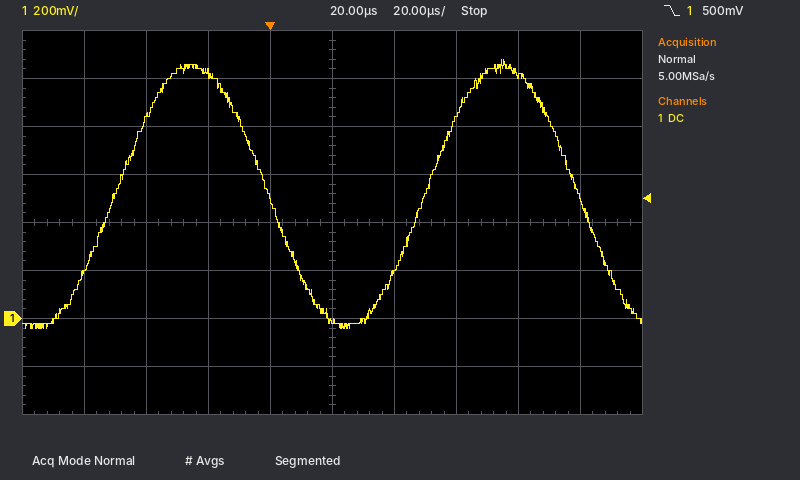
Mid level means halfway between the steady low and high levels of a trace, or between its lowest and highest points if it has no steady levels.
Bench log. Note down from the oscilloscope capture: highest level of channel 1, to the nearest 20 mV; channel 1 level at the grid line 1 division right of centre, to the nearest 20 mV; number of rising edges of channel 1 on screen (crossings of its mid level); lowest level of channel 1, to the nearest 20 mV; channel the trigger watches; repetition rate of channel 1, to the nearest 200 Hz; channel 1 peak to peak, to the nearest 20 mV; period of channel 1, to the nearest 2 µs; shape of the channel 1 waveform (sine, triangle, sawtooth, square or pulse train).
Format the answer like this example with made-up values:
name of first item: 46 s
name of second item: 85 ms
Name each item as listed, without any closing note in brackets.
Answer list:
highest level of channel 1, to the nearest 20 mV: 1.08 V
channel 1 level at the grid line 1 division right of centre, to the nearest 20 mV: 200 mV
number of rising edges of channel 1 on screen: 2
lowest level of channel 1, to the nearest 20 mV: -40 mV
channel the trigger watches: channel 1
repetition rate of channel 1, to the nearest 200 Hz: 10.0 kHz
channel 1 peak to peak, to the nearest 20 mV: 1.12 V
period of channel 1, to the nearest 2 µs: 100 µs
shape of the channel 1 waveform: sine
